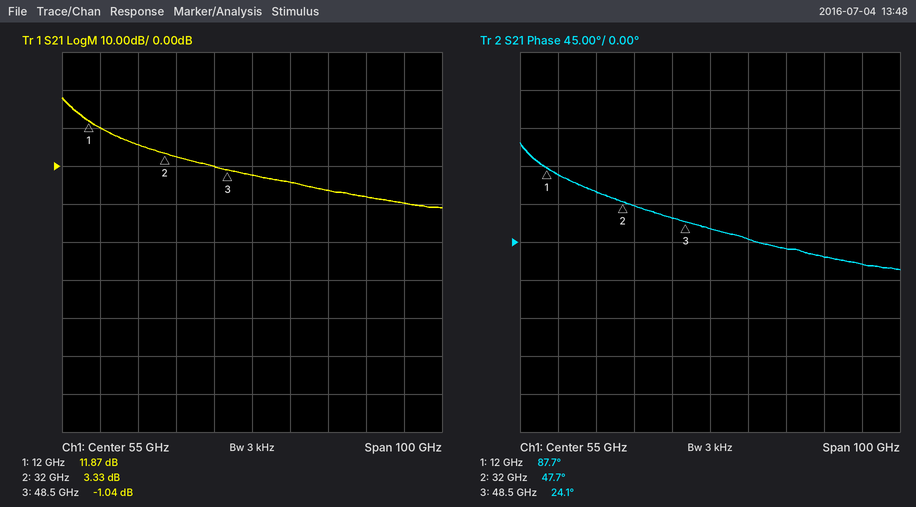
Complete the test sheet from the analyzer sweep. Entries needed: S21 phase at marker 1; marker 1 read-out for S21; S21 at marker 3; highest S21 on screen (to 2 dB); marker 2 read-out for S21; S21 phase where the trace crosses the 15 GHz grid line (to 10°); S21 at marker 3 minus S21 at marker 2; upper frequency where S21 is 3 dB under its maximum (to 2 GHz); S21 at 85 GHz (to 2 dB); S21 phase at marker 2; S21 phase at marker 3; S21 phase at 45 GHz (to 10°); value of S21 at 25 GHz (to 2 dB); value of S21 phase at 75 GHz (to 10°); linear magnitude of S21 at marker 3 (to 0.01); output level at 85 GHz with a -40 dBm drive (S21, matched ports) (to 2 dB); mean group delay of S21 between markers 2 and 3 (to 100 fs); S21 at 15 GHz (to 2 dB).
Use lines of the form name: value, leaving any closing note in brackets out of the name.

S21 phase at marker 1: 87.7°
marker 1 read-out for S21: 11.87 dB
S21 at marker 3: -1.04 dB
highest S21 on screen: 18 dB
marker 2 read-out for S21: 3.33 dB
S21 phase where the trace crosses the 15 GHz grid line: 80°
S21 at marker 3 minus S21 at marker 2: -4.37 dB
upper frequency where S21 is 3 dB under its maximum: 8 GHz
S21 at 85 GHz: -8 dB
S21 phase at marker 2: 47.7°
S21 phase at marker 3: 24.1°
S21 phase at 45 GHz: 30°
value of S21 at 25 GHz: 6 dB
value of S21 phase at 75 GHz: -10°
linear magnitude of S21 at marker 3: 0.89
output level at 85 GHz with a -40 dBm drive (S21, matched ports): -48 dBm
mean group delay of S21 between markers 2 and 3: 4.0 ps
S21 at 15 GHz: 10 dB
